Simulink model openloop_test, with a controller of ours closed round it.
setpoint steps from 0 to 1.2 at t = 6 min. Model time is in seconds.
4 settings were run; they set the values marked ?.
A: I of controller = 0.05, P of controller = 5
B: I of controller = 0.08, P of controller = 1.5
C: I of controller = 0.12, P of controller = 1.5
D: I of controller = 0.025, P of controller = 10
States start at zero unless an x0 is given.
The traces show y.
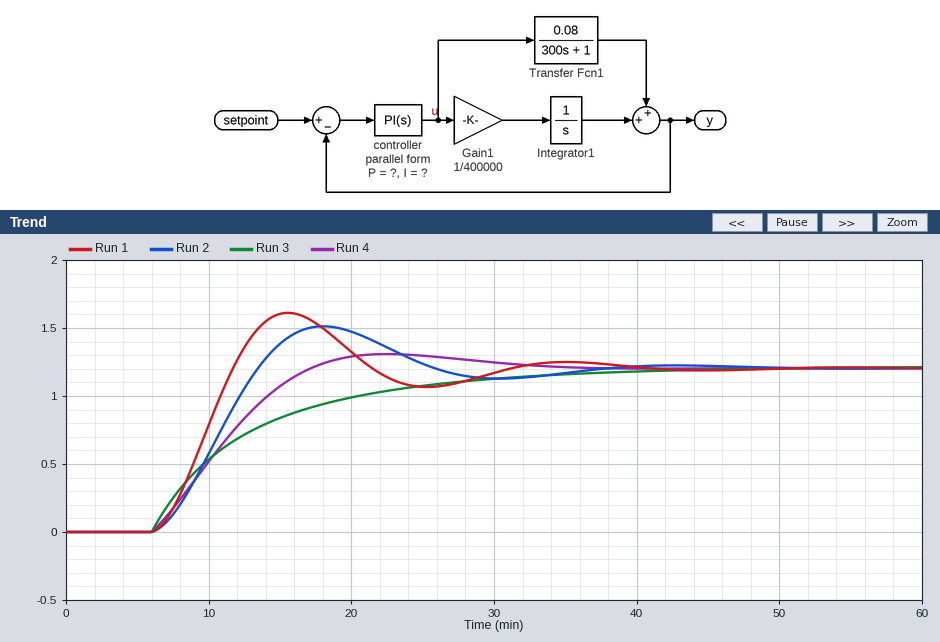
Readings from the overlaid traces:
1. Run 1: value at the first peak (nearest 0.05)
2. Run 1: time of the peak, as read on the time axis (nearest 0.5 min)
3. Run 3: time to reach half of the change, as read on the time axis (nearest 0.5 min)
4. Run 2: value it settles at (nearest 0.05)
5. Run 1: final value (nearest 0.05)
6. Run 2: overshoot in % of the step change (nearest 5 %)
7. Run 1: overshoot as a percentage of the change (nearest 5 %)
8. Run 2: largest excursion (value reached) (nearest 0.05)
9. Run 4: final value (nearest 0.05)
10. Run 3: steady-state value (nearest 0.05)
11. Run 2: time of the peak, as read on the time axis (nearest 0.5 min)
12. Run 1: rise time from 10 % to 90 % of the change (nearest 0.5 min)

1.60
15.5 min
11.0 min
1.20
1.20
25 %
35 %
1.50
1.20
1.20
18.0 min
4.0 min
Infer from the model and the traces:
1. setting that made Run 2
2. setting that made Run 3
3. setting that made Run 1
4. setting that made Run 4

B
D
C
A
